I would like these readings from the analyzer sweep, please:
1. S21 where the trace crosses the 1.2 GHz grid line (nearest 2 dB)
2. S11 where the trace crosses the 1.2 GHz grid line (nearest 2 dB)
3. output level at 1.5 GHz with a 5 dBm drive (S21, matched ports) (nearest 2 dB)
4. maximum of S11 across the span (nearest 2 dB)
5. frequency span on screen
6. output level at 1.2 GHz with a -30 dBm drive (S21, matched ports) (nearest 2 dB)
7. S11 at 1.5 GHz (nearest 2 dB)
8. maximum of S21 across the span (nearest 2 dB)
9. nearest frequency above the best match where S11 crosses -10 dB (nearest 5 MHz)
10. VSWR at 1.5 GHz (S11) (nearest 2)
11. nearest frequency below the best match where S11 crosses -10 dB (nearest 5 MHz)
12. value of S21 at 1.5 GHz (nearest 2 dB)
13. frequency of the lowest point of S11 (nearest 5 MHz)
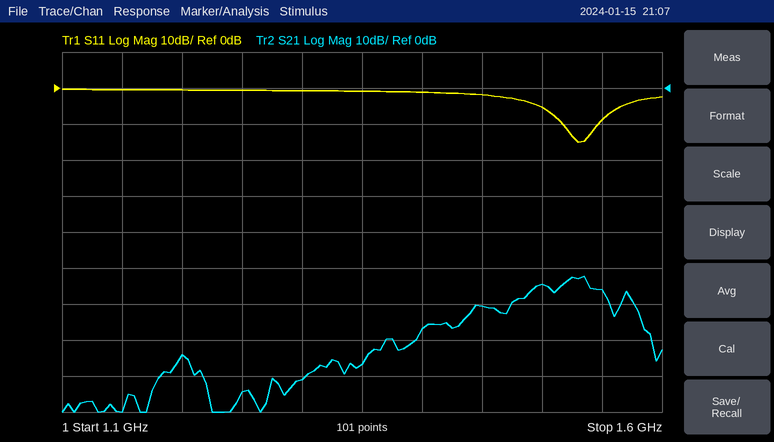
-74 dB
0 dB
-50 dBm
0 dB
500 MHz
-104 dBm
-6 dB
-52 dB
1.545 GHz
4
1.515 GHz
-54 dB
1.530 GHz
